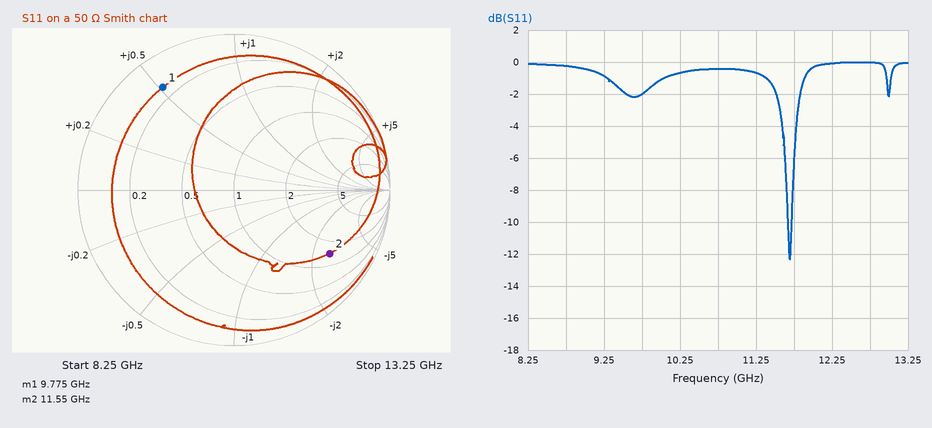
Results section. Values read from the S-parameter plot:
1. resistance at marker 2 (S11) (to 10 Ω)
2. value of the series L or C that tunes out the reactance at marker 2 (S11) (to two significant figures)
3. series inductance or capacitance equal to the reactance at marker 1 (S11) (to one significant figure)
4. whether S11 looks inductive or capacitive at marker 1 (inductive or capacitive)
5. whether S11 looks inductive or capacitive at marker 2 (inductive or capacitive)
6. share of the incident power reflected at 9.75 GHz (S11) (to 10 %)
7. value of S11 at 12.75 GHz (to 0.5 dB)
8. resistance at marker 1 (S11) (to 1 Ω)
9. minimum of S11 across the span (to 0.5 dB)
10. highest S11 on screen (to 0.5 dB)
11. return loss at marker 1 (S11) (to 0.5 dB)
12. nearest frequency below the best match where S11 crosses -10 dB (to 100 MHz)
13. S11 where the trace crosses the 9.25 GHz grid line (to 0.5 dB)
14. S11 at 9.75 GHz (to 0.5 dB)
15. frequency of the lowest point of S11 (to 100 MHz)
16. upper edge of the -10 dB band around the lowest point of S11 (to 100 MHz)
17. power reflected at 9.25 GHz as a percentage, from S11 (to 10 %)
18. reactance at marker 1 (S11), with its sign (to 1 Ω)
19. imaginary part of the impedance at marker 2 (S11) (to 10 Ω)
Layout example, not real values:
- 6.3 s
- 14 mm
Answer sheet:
- 70 Ω
- 1.8 nH
- 400 pH
- inductive
- capacitive
- 60 %
- 0.0 dB
- 7 Ω
- -12.5 dB
- 0.0 dB
- 2.0 dB
- 11.7 GHz
- -1.0 dB
- -2.0 dB
- 11.7 GHz
- 11.7 GHz
- 80 %
- +26 Ω
- -130 Ω
